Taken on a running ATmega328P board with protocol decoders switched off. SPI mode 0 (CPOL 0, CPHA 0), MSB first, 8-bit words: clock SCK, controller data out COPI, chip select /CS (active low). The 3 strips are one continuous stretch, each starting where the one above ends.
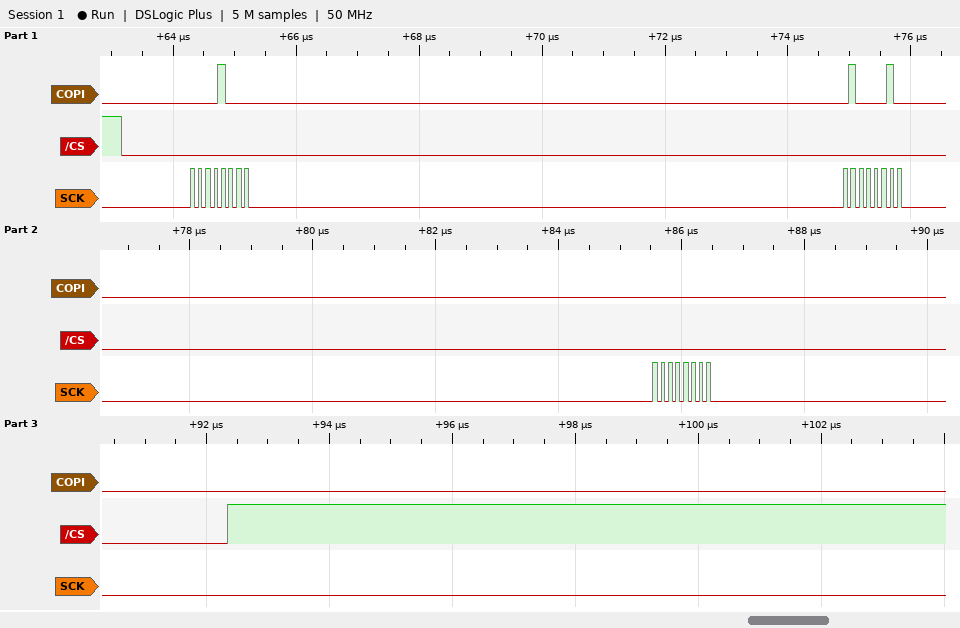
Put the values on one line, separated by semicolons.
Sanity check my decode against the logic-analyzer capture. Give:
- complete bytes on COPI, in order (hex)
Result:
0x08 0x42 0x00
